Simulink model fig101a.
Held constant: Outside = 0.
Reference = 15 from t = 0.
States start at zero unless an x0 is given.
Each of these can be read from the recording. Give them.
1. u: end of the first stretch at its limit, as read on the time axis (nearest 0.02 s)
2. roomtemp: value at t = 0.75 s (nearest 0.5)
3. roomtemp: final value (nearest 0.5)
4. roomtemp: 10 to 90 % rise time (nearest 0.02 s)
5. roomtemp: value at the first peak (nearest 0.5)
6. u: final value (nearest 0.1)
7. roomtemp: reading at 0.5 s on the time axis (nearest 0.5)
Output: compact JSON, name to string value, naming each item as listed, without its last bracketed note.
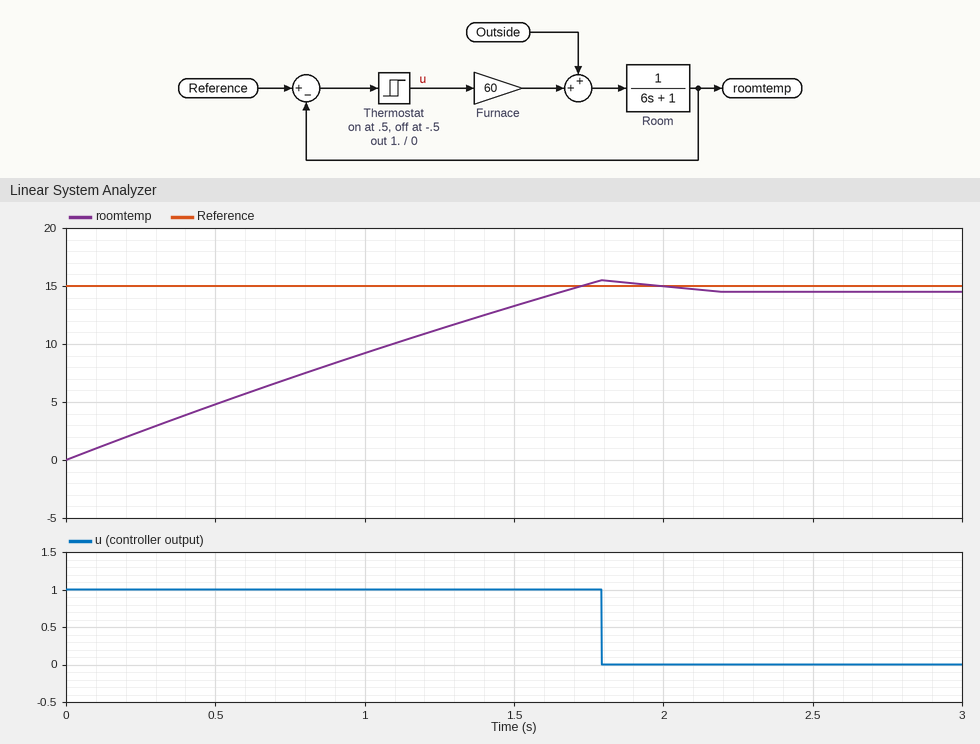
{"u: end of the first stretch at its limit, as read on the time axis": "1.80 s", "roomtemp: value at t = 0.75 s": "7.0", "roomtemp: final value": "14.5", "roomtemp: 10 to 90 % rise time": "1.32 s", "roomtemp: value at the first peak": "15.5", "u: final value": "0.0", "roomtemp: reading at 0.5 s on the time axis": "5.0"}
